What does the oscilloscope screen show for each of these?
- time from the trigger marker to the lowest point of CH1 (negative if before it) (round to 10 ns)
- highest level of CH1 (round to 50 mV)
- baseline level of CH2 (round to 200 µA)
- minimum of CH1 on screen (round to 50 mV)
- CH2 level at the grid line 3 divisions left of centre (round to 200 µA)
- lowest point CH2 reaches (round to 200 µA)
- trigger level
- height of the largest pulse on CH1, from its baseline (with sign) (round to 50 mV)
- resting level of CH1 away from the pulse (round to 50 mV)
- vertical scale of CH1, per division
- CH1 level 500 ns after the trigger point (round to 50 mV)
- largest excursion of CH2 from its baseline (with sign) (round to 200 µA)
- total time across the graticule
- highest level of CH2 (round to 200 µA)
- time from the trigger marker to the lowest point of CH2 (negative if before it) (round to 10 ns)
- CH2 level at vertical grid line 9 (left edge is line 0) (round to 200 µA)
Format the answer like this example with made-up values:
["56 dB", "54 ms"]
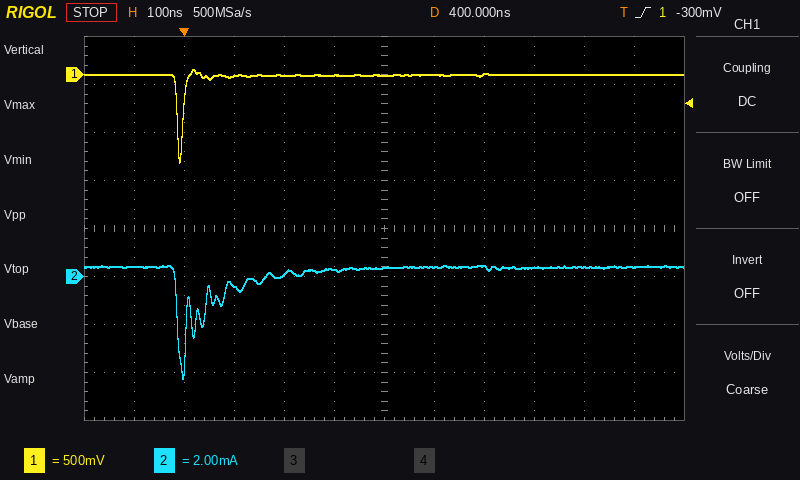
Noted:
["-10 ns", "50 mV", "400 µA", "-900 mV", "-400 µA", "-4.2 mA", "-300 mV", "-900 mV", "0 mV", "500 mV", "0 mV", "-4.6 mA", "1.2 µs", "400 µA", "0 ns", "400 µA"]
